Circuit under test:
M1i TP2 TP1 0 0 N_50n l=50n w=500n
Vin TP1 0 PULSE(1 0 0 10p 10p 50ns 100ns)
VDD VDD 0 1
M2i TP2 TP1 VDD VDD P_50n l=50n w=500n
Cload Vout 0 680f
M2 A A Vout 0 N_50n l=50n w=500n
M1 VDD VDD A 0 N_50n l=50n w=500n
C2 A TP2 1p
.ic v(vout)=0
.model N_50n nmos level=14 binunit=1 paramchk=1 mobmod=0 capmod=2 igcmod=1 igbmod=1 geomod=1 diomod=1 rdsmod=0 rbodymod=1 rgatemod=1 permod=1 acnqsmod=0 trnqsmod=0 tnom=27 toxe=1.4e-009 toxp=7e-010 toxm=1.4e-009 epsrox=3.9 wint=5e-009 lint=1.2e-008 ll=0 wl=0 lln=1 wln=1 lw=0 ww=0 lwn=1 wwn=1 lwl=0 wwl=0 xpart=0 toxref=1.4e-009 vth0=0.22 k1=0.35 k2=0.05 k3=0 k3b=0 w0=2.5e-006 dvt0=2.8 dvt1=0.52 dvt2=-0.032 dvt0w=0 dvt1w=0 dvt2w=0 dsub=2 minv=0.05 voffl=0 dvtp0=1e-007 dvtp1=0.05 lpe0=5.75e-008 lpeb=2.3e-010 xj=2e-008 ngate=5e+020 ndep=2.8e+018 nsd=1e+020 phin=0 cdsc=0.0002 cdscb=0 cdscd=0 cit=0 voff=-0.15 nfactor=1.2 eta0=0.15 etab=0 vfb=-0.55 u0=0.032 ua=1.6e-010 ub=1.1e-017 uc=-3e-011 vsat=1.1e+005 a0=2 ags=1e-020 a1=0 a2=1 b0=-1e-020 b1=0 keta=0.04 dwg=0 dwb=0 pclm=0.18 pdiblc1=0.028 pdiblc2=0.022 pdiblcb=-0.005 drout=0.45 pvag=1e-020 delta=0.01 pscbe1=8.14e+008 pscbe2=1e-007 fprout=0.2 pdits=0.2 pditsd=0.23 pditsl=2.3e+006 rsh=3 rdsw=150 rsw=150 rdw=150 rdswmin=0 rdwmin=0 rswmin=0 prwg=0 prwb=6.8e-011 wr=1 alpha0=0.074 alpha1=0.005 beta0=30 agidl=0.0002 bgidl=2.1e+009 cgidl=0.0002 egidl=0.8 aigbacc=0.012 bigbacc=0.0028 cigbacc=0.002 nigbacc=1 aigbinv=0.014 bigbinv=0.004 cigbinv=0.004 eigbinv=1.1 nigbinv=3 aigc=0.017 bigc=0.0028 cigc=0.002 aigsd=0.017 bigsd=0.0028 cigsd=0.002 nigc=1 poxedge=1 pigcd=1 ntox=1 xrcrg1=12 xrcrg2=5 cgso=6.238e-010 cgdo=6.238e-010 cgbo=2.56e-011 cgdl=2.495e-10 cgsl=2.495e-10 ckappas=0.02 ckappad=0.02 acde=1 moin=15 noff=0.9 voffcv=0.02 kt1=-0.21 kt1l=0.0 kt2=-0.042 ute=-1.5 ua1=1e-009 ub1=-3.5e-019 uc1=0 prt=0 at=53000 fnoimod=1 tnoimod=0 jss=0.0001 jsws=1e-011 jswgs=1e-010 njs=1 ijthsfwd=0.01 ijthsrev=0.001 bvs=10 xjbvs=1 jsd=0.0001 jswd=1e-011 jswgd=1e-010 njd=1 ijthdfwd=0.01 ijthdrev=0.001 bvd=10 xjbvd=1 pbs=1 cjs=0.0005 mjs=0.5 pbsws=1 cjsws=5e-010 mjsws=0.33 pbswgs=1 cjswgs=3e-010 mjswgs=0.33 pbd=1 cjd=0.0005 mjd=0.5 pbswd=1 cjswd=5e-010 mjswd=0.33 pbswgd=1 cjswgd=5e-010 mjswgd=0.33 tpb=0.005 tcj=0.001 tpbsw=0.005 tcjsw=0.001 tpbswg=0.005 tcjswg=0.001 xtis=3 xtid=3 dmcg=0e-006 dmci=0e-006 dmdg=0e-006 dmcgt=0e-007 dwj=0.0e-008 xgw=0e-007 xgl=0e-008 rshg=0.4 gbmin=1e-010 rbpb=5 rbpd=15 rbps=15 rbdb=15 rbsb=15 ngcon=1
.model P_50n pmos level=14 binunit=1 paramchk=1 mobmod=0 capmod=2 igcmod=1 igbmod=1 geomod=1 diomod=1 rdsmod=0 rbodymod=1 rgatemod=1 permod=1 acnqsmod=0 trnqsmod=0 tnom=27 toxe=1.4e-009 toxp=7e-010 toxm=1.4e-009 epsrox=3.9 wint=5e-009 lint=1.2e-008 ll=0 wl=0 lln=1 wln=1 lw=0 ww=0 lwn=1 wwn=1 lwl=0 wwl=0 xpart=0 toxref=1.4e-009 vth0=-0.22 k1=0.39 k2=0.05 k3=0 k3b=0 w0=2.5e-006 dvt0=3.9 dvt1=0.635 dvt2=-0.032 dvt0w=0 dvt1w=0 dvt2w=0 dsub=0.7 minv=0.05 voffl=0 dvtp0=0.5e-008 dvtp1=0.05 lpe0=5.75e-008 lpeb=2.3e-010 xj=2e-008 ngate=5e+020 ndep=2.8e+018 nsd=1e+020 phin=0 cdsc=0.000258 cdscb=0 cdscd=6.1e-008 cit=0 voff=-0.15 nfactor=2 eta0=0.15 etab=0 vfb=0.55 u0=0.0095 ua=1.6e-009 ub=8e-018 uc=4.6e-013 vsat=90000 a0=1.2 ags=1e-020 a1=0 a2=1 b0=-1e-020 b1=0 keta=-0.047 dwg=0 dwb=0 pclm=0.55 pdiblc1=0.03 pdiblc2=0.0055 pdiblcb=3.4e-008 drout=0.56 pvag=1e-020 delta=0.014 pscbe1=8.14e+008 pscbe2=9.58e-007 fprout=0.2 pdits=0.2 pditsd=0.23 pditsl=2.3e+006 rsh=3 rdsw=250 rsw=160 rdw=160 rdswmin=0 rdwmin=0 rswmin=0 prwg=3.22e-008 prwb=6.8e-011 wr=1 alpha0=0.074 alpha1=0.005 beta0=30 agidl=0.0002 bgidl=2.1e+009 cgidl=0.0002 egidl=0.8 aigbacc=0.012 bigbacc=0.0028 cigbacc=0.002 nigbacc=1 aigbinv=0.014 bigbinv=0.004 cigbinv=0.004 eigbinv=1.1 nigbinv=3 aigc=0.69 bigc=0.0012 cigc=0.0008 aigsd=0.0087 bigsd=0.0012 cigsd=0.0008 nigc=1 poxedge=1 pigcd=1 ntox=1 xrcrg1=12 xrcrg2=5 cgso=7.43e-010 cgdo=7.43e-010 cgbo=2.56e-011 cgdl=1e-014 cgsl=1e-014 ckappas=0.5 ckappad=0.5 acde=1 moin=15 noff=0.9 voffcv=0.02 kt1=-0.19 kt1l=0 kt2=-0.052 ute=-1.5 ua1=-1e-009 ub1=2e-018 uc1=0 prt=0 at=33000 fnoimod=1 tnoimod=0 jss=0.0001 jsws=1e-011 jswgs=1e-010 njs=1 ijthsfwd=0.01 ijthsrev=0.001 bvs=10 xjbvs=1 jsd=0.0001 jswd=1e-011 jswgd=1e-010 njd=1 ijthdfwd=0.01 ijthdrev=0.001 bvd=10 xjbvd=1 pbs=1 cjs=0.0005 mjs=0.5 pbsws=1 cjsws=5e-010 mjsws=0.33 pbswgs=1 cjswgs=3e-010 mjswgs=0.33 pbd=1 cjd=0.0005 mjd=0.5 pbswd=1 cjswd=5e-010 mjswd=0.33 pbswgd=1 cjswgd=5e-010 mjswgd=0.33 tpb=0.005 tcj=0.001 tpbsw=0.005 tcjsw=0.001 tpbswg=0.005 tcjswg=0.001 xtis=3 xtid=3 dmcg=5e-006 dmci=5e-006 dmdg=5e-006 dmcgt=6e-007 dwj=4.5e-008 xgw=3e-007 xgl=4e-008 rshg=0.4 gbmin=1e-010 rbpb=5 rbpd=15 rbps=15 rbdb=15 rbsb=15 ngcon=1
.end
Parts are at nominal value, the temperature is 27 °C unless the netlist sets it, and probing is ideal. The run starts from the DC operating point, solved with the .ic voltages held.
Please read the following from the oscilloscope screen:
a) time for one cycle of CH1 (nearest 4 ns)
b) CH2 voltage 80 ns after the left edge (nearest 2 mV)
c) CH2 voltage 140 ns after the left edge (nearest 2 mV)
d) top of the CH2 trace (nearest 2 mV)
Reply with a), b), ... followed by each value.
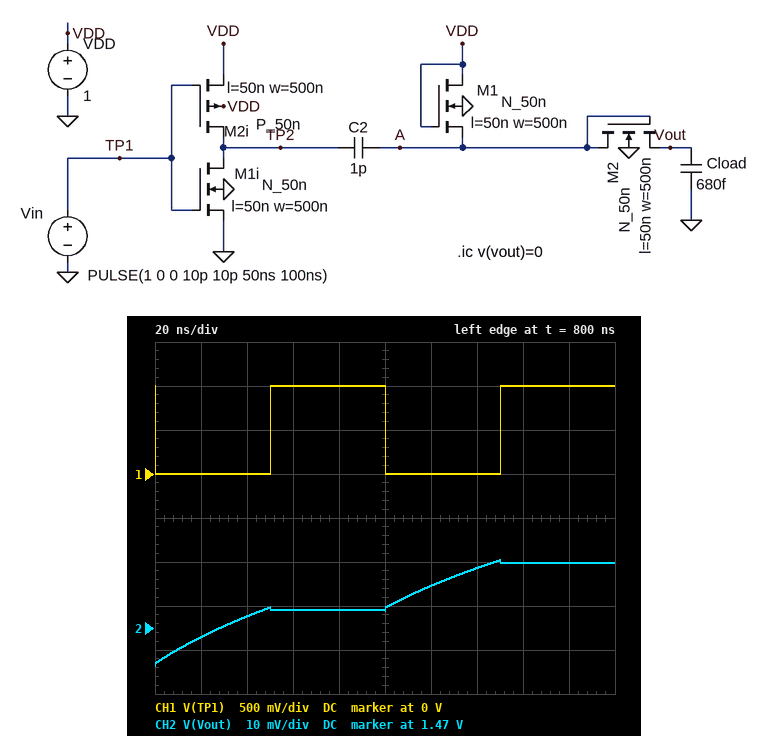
a) 100 ns
b) 1.474 V
c) 1.484 V
d) 1.486 V
